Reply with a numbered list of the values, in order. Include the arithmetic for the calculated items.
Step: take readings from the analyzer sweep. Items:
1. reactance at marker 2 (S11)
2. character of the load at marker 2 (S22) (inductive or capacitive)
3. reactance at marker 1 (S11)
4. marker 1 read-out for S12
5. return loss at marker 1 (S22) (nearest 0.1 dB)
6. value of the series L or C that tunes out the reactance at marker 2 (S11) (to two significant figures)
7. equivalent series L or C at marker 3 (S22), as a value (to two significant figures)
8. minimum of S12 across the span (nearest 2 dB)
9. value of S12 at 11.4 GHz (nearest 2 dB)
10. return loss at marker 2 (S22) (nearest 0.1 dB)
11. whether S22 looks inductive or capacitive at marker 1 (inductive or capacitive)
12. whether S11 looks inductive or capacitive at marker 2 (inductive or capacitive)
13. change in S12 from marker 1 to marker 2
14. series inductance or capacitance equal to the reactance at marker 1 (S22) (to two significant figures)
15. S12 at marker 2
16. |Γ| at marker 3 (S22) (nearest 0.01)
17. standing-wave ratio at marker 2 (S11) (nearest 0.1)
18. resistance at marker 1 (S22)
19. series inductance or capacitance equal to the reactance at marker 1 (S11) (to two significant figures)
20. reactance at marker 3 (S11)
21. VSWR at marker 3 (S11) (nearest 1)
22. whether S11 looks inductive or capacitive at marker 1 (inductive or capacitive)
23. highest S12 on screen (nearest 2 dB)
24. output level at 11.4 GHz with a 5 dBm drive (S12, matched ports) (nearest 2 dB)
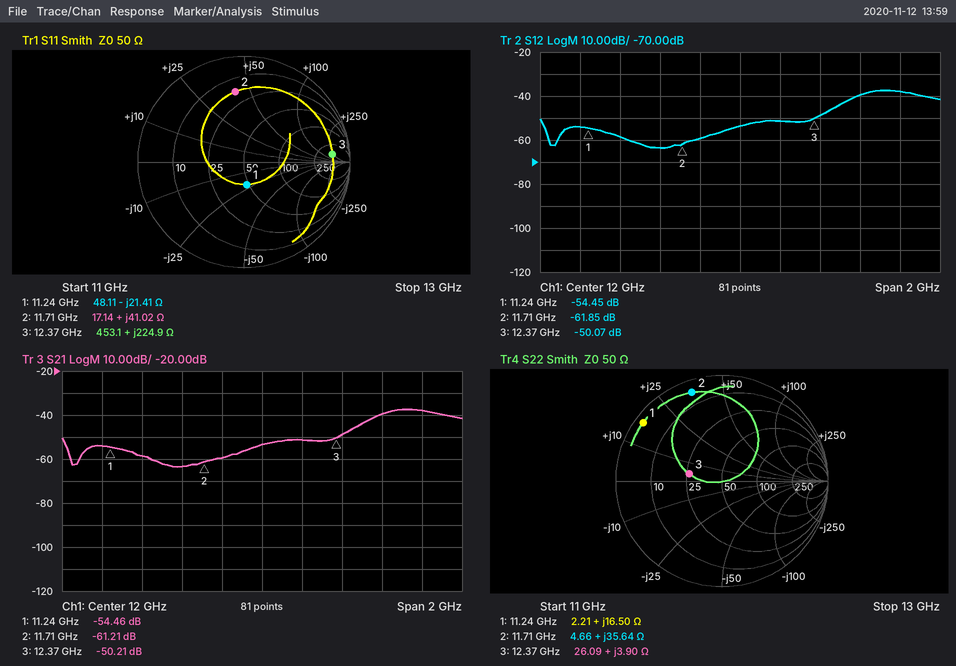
1. +41.02 Ω
2. inductive
3. -21.41 Ω
4. -54.45 dB
5. 0.7 dB
6. C = 1/(2π × 11.71 GHz × 41.02 Ω) ≈ 331 fF, so 330 fF to two significant figures
7. L = 3.9 Ω/(2π × 12.37 GHz) ≈ 50 pH
8. -64 dB
9. -58 dB
10. 1.1 dB
11. inductive
12. inductive
13. -61.85 − (-54.45) = -7.40 dB
14. L = 16.5 Ω/(2π × 11.24 GHz) ≈ 234 pH, so 230 pH to two significant figures
15. -61.85 dB
16. 0.32
17. 5.0
18. 2.21 Ω
19. C = 1/(2π × 11.24 GHz × 21.41 Ω) ≈ 661 fF, so 660 fF to two significant figures
20. +224.9 Ω
21. 11
22. capacitive
23. -38 dB
24. 5 dBm + (-58 dB) = -54 dBm
